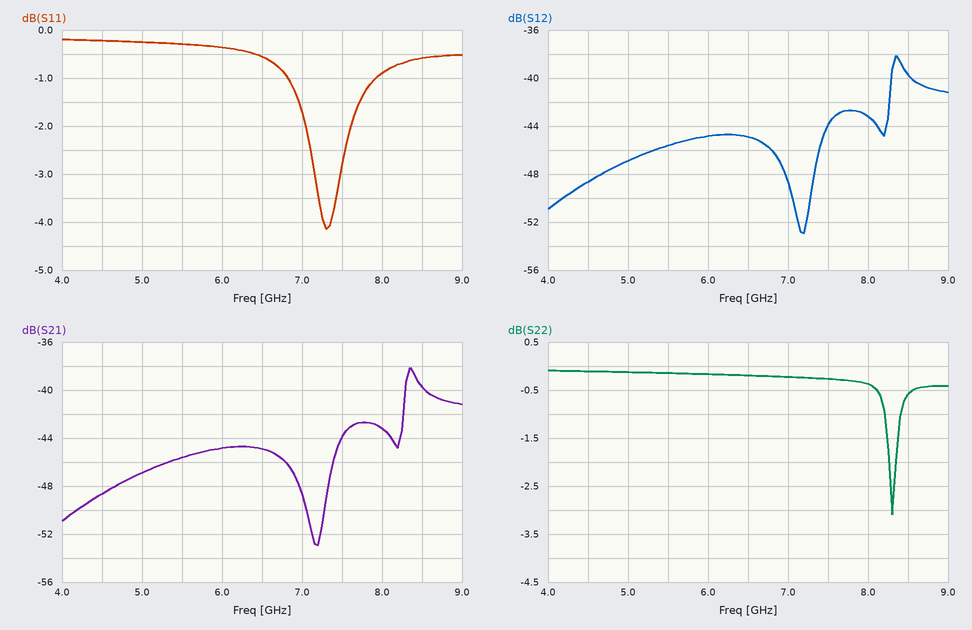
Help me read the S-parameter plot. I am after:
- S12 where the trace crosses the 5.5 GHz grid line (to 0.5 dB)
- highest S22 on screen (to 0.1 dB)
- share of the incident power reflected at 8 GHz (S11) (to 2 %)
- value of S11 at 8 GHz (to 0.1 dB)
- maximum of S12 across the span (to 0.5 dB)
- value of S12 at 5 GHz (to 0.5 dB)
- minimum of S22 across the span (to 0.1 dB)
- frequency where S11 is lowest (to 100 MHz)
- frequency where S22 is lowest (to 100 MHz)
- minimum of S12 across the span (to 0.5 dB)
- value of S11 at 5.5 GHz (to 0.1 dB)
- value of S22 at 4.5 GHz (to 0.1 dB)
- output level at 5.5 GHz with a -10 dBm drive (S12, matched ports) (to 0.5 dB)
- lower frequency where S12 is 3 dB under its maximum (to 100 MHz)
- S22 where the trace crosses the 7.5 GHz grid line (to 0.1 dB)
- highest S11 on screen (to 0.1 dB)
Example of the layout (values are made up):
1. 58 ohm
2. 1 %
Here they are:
1. -45.5 dB
2. -0.1 dB
3. 82 %
4. -0.9 dB
5. -38.0 dB
6. -47.0 dB
7. -3.1 dB
8. 7.3 GHz
9. 8.3 GHz
10. -53.0 dB
11. -0.3 dB
12. -0.1 dB
13. -55.5 dBm
14. 8.3 GHz
15. -0.3 dB
16. -0.2 dB
